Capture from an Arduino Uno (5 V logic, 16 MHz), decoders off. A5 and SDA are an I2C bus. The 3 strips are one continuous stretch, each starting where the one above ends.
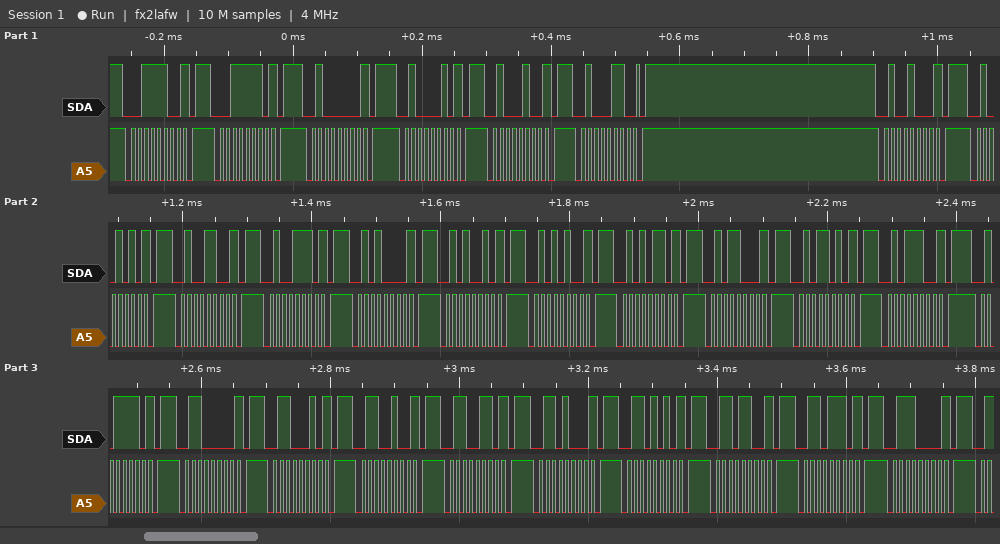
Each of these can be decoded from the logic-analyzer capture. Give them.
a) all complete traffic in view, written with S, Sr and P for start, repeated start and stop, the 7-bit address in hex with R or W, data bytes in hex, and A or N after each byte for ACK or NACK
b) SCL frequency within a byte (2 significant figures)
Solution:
S 1EW N P S 1FW N P S 20W N P S 21W N P S 22W N P S 23W A P S 24W N P S 25W N P S 26W N P S 27W N P S 28W N P S 29W N P S 2AW N P S 2BW N P S 2CW N P S 2DW N P S 2EW N P S 2FW N P S 30W N P S 31W N P S 32W N P S 33W N P S 34W N P S 35W N P S 36W N P S 37W N P S 38W N P
100 kHz
